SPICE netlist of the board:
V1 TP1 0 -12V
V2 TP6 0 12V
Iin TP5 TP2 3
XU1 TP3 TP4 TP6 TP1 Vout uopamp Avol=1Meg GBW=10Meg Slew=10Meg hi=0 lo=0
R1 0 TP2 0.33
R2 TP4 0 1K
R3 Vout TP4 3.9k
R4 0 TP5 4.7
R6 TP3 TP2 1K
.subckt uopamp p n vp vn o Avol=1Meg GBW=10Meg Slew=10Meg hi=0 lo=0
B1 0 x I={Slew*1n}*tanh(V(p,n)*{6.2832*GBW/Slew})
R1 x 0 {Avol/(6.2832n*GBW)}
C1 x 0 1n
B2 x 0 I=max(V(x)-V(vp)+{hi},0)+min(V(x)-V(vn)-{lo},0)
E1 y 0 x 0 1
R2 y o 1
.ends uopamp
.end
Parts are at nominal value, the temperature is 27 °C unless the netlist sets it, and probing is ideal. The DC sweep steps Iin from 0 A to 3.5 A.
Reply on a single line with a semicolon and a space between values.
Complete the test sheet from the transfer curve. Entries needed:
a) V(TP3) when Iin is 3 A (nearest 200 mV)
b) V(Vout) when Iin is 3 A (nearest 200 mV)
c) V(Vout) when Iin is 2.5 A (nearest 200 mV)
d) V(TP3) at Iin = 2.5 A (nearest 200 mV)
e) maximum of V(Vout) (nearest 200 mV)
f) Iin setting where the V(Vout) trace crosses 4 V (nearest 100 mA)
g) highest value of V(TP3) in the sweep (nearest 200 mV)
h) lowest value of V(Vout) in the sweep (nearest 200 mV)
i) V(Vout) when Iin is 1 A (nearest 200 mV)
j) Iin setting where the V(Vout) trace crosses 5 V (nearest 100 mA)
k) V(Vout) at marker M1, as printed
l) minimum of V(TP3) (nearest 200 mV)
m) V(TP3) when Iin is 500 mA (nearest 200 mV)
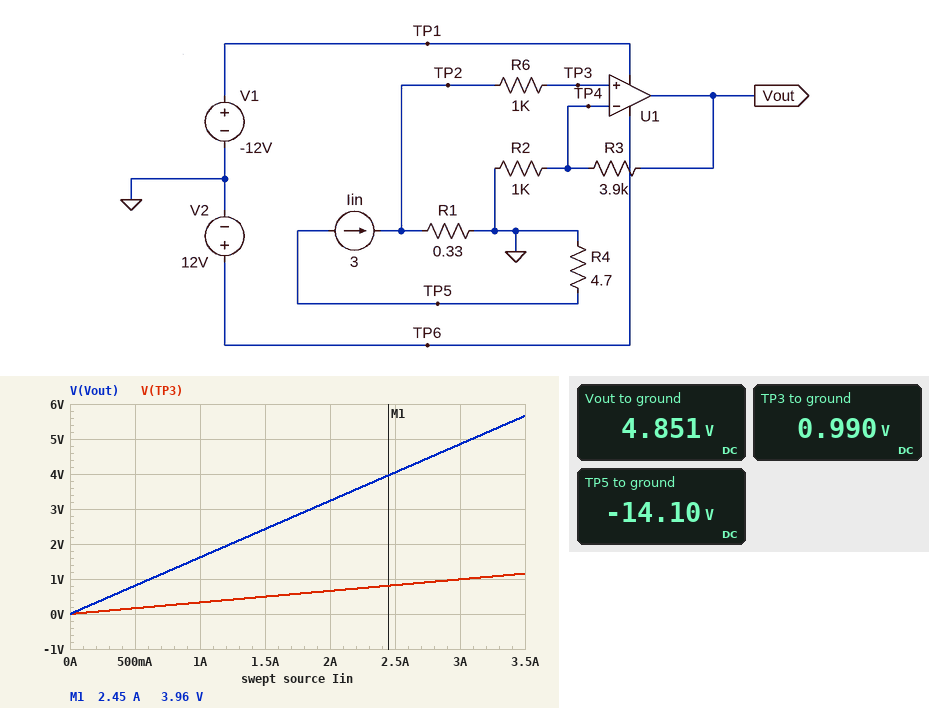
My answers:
1.0 V; 4.8 V; 4.0 V; 800 mV; 5.6 V; 2.5 A; 1.2 V; 0 V; 1.6 V; 3.1 A; 3.96 V; 0 V; 200 mV
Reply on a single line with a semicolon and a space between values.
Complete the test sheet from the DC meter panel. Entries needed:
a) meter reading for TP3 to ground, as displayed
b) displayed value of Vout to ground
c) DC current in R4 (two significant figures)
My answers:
0.990 V; 4.851 V; 3.0 A
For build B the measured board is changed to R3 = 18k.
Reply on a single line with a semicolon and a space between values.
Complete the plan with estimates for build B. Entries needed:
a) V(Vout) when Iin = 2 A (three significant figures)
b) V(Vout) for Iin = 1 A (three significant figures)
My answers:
12.0 V; 6.27 V
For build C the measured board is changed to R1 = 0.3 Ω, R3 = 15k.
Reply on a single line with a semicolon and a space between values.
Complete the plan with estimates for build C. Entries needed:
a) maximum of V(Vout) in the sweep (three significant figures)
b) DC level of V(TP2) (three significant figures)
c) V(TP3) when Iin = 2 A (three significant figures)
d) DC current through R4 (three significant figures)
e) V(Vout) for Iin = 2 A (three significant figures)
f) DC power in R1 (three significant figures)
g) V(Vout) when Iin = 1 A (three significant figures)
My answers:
12.0 V; 900 mV; 600 mV; 3.00 A; 9.60 V; 2.70 W; 4.80 V
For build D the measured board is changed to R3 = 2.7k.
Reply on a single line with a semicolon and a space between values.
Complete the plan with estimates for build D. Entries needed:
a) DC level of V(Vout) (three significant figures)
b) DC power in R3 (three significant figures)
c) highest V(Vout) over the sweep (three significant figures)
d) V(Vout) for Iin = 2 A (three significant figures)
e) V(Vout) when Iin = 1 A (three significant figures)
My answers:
3.66 V; 2.65 mW; 4.27 V; 2.44 V; 1.22 V
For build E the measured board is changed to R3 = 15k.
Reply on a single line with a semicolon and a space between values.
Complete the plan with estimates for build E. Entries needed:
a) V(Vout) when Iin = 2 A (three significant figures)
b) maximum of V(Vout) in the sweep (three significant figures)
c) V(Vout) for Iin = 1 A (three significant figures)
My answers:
10.6 V; 12.0 V; 5.28 V
